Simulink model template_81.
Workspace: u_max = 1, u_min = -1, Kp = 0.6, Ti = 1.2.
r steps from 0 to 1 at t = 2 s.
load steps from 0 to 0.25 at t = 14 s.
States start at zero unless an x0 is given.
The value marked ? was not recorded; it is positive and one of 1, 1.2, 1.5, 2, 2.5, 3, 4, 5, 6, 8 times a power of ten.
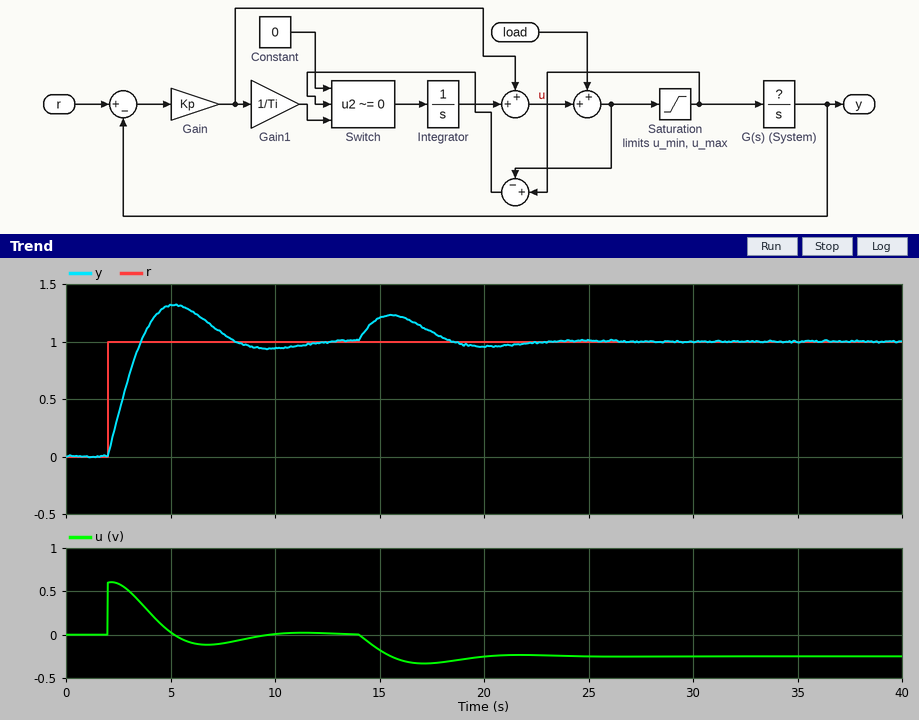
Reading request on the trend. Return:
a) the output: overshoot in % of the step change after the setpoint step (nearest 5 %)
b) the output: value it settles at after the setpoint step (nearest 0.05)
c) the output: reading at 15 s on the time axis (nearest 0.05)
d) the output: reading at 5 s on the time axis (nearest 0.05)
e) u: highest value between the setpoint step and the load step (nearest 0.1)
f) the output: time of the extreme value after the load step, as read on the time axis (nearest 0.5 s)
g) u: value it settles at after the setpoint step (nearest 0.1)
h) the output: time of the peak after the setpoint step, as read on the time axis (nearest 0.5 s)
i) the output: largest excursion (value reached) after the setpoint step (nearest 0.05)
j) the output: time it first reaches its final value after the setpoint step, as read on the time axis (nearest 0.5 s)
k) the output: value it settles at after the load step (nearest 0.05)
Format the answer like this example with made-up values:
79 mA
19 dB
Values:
30 %
1.00
1.20
1.30
0.6
15.5 s
0.0
5.0 s
1.30
3.5 s
1.00
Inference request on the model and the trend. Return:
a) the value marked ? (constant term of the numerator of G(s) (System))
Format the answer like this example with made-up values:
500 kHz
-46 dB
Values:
1.2
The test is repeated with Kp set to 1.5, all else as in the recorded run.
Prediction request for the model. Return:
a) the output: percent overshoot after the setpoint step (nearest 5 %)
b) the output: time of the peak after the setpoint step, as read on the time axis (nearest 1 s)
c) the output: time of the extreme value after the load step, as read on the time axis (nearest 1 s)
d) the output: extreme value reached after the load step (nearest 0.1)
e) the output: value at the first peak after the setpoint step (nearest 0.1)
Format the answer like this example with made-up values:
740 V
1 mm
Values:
15 %
4 s
15 s
1.1
1.1
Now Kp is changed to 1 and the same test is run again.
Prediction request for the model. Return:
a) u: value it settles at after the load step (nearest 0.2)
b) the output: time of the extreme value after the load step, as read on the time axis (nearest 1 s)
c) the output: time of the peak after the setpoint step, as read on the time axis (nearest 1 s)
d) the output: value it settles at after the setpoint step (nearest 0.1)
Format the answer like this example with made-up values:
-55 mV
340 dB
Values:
-0.2
15 s
4 s
1.0
